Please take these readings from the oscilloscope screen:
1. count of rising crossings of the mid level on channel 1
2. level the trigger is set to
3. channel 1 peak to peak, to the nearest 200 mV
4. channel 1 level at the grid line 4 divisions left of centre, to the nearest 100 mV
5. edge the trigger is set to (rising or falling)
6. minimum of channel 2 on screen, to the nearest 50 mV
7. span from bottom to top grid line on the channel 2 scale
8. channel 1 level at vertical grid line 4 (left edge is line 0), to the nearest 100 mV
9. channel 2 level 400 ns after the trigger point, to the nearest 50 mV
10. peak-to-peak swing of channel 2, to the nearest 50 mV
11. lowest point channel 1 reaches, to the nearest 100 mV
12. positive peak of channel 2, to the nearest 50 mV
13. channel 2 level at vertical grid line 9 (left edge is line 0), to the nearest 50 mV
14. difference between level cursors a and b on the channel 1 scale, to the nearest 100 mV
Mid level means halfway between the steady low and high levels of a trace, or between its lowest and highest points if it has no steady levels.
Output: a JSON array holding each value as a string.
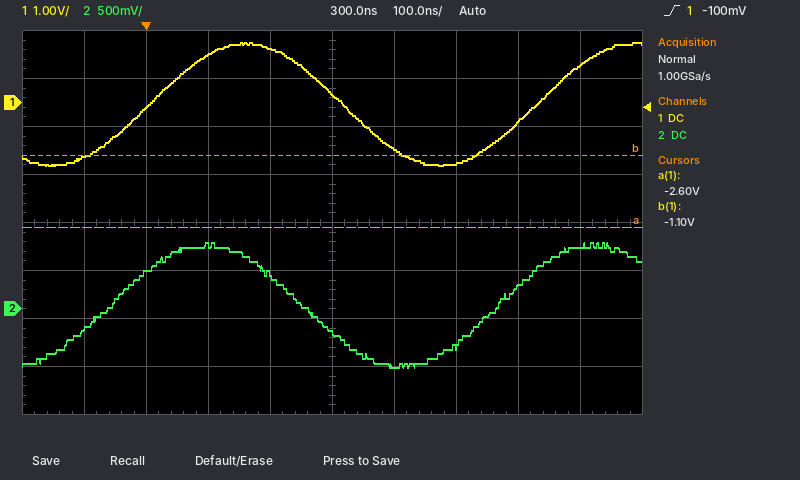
["2", "-100 mV", "2.6 V", "-1.1 V", "rising", "-600 mV", "4 V", "1.1 V", "-600 mV", "1.30 V", "-1.3 V", "700 mV", "650 mV", "1.5 V"]
